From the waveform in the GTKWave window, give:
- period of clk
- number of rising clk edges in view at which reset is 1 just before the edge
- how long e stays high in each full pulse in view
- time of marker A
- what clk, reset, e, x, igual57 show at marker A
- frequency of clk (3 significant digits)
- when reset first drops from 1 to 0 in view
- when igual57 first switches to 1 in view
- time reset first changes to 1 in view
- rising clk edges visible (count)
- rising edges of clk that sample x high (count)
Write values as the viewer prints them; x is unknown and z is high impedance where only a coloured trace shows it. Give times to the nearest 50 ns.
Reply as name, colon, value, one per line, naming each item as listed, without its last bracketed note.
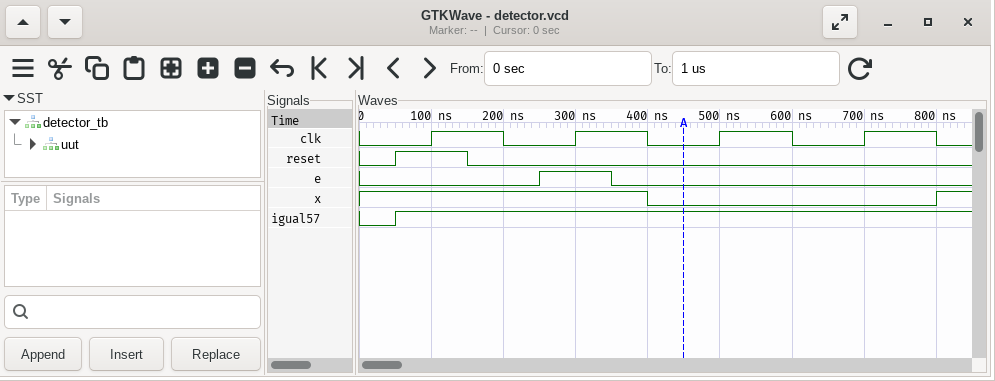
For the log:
period of clk: 200 ns
number of rising clk edges in view at which reset is 1 just before the edge: 1
how long e stays high in each full pulse in view: 100 ns
time of marker A: 450 ns
what clk, reset, e, x, igual57 show at marker A: clk=0, reset=0, e=0, x=0, igual57=1
frequency of clk: 5.00 MHz
when reset first drops from 1 to 0 in view: 150 ns
when igual57 first switches to 1 in view: 50 ns
time reset first changes to 1 in view: 50 ns
rising clk edges visible: 4
rising edges of clk that sample x high: 2
